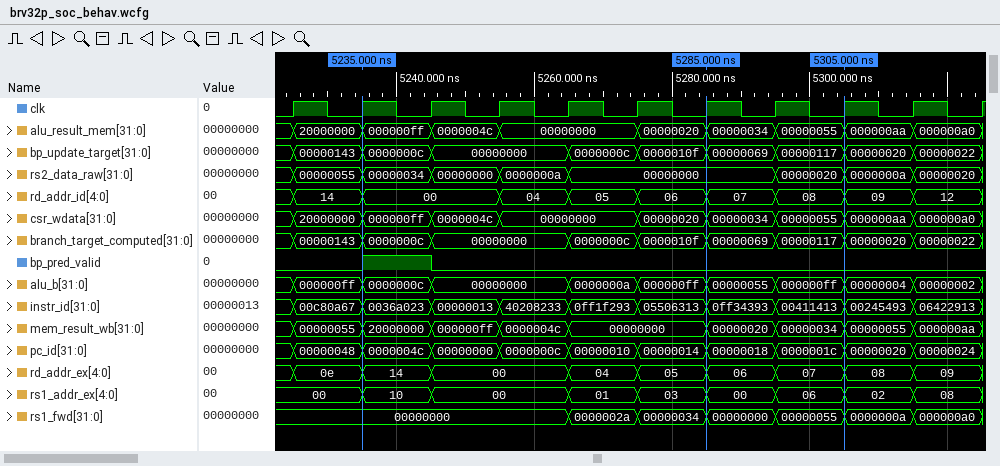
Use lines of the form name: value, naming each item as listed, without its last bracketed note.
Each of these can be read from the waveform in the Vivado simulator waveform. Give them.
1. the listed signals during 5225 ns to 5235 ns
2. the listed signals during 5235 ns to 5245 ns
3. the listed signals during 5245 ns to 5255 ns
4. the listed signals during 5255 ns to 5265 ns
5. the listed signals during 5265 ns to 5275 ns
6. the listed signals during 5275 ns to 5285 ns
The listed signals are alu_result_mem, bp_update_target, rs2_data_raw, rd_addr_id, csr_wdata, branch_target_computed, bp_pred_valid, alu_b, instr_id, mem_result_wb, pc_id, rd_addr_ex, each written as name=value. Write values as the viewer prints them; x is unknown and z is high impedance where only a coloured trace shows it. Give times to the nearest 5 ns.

the listed signals during 5225 ns to 5235 ns: alu_result_mem=20000000, bp_update_target=00000143, rs2_data_raw=00000055, rd_addr_id=14, csr_wdata=20000000, branch_target_computed=00000143, bp_pred_valid=0, alu_b=000000ff, instr_id=00c80a67, mem_result_wb=00000055, pc_id=00000048, rd_addr_ex=0e
the listed signals during 5235 ns to 5245 ns: alu_result_mem=000000ff, bp_update_target=0000000c, rs2_data_raw=00000034, rd_addr_id=00, csr_wdata=000000ff, branch_target_computed=0000000c, bp_pred_valid=1, alu_b=0000000c, instr_id=0036a023, mem_result_wb=20000000, pc_id=0000004c, rd_addr_ex=14
the listed signals during 5245 ns to 5255 ns: alu_result_mem=0000004c, bp_update_target=00000000, rs2_data_raw=00000000, rd_addr_id=00, csr_wdata=0000004c, branch_target_computed=00000000, bp_pred_valid=0, alu_b=00000000, instr_id=00000013, mem_result_wb=000000ff, pc_id=00000000, rd_addr_ex=00
the listed signals during 5255 ns to 5265 ns: alu_result_mem=00000000, bp_update_target=00000000, rs2_data_raw=0000000a, rd_addr_id=04, csr_wdata=00000000, branch_target_computed=00000000, bp_pred_valid=0, alu_b=00000000, instr_id=40208233, mem_result_wb=0000004c, pc_id=0000000c, rd_addr_ex=00
the listed signals during 5265 ns to 5275 ns: alu_result_mem=00000000, bp_update_target=0000000c, rs2_data_raw=00000000, rd_addr_id=05, csr_wdata=00000000, branch_target_computed=0000000c, bp_pred_valid=0, alu_b=0000000a, instr_id=0ff1f293, mem_result_wb=00000000, pc_id=00000010, rd_addr_ex=04
the listed signals during 5275 ns to 5285 ns: alu_result_mem=00000020, bp_update_target=0000010f, rs2_data_raw=00000000, rd_addr_id=06, csr_wdata=00000020, branch_target_computed=0000010f, bp_pred_valid=0, alu_b=000000ff, instr_id=05506313, mem_result_wb=00000000, pc_id=00000014, rd_addr_ex=05
